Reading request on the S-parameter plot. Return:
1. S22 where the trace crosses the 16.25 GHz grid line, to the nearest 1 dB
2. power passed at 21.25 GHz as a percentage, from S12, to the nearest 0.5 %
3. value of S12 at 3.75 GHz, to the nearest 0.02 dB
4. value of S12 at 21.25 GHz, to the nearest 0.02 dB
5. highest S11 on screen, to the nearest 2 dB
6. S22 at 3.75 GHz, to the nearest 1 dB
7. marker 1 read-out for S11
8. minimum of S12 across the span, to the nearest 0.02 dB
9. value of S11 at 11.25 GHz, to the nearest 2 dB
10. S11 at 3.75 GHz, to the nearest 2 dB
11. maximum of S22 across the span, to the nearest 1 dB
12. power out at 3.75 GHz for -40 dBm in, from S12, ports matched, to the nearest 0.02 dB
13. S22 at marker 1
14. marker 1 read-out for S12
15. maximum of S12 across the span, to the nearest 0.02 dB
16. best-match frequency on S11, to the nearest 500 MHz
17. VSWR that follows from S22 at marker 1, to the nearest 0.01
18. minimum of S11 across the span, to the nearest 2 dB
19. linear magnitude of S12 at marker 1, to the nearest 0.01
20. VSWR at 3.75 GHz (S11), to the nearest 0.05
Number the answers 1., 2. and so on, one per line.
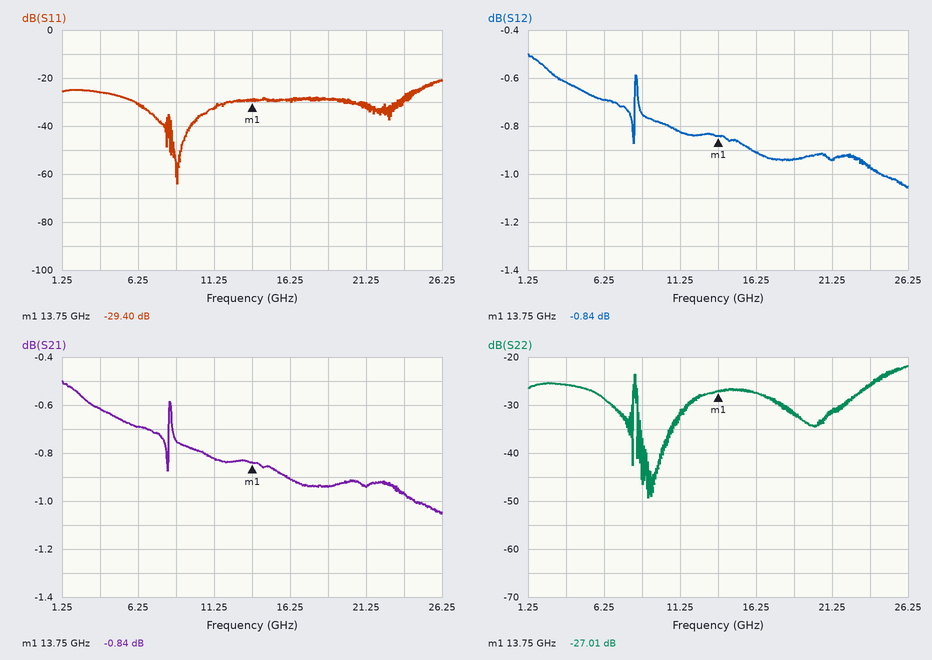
1. -27 dB
2. 80.5 %
3. -0.62 dB
4. -0.94 dB
5. -20 dB
6. -26 dB
7. -29.40 dB
8. -1.06 dB
9. -32 dB
10. -26 dB
11. -22 dB
12. -40.62 dBm
13. -27.01 dB
14. -0.84 dB
15. -0.50 dB
16. 9.0 GHz
17. 1.09
18. -64 dB
19. 0.91
20. 1.10
